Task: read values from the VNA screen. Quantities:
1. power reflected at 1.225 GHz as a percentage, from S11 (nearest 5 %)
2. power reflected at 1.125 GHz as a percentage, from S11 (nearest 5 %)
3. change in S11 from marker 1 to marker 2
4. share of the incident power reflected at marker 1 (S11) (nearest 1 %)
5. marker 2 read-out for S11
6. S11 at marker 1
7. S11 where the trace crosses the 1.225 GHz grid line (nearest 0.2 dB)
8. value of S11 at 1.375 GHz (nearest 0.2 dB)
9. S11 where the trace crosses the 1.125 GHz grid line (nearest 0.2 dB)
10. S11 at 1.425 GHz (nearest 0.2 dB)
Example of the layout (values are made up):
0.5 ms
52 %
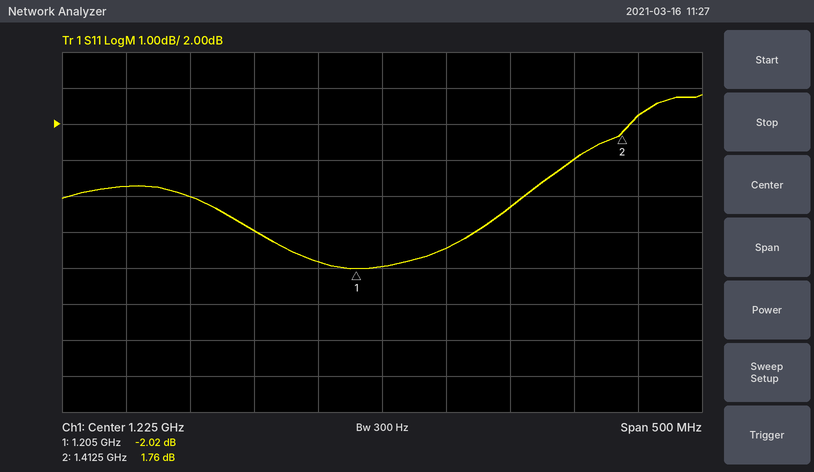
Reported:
65 %
80 %
3.78 dB
63 %
1.76 dB
-2.02 dB
-2.0 dB
1.0 dB
-1.0 dB
2.2 dB
